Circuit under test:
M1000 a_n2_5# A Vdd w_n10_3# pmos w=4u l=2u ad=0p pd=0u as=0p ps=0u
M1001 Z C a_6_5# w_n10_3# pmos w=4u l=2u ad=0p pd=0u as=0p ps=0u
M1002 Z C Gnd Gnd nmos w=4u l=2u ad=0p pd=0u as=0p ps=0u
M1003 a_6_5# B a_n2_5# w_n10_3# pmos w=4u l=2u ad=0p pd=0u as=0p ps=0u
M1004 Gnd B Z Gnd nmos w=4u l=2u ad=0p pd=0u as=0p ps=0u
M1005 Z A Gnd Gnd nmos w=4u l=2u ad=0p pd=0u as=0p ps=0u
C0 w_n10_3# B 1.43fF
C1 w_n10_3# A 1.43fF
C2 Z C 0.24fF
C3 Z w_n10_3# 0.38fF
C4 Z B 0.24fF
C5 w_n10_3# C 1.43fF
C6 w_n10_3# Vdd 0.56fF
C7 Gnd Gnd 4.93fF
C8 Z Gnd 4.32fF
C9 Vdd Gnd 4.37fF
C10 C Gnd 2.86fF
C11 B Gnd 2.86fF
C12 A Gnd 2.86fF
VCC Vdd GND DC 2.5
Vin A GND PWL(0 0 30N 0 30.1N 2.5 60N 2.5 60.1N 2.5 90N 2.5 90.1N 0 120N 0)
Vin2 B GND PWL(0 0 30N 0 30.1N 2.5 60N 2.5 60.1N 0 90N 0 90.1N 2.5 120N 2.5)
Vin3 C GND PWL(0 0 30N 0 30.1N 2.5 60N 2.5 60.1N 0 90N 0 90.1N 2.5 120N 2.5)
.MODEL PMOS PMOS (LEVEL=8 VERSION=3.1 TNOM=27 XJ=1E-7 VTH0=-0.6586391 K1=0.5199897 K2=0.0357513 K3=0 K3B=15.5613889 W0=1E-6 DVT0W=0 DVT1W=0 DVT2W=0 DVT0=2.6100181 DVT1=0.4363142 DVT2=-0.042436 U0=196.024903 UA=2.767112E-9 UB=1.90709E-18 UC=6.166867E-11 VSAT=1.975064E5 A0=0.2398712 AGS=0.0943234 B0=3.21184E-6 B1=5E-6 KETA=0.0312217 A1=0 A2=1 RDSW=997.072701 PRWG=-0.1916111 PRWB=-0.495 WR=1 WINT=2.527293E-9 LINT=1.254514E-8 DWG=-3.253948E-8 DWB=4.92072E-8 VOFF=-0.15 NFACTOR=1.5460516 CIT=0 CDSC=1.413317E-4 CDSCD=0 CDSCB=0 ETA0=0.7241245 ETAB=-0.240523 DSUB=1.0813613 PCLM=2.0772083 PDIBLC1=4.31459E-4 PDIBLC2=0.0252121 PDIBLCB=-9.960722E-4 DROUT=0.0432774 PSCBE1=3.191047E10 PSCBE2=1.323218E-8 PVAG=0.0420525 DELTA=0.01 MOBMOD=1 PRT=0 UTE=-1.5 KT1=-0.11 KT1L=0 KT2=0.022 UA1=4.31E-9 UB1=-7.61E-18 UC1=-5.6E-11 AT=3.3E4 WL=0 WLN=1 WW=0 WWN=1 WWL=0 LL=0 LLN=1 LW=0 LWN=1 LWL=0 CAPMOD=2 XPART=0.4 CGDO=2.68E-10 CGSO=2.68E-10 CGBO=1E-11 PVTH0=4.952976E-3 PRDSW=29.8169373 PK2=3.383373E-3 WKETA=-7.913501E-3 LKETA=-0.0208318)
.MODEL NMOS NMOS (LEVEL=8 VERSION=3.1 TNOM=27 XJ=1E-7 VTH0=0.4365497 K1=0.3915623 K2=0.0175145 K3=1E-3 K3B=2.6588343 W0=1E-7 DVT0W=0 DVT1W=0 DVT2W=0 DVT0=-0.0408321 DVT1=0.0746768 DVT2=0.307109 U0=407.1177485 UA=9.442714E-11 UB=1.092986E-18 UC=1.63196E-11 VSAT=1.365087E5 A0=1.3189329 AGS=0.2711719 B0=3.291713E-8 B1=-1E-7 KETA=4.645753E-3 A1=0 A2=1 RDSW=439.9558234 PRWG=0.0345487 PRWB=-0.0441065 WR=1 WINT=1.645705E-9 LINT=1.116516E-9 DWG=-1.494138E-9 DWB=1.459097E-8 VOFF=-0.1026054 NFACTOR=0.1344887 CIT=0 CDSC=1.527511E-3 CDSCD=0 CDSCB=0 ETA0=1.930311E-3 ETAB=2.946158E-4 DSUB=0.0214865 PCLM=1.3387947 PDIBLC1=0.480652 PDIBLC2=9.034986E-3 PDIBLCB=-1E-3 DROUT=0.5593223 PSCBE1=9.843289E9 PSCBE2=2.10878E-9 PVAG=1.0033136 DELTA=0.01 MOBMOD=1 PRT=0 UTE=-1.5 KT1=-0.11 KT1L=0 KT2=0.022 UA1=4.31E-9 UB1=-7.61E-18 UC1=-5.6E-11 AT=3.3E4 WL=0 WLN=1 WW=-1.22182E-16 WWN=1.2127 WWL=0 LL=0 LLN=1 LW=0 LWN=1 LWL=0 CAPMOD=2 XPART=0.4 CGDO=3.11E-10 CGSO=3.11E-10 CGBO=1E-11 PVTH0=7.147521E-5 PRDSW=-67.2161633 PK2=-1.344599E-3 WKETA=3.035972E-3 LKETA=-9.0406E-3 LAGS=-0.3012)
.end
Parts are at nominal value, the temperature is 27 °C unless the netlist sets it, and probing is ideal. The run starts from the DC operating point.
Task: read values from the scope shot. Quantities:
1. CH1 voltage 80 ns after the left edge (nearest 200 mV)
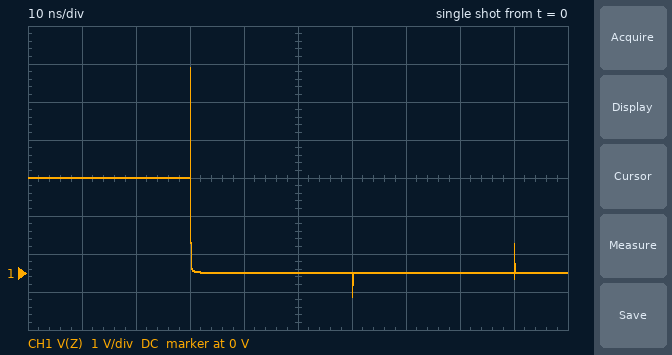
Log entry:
0 V
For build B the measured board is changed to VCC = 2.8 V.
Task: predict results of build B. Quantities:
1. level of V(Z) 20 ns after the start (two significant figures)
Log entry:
2.8 V
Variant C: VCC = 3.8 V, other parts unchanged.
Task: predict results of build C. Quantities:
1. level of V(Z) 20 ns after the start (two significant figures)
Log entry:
3.8 V
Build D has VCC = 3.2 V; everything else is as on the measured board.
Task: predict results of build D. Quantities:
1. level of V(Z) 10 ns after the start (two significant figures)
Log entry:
3.2 V
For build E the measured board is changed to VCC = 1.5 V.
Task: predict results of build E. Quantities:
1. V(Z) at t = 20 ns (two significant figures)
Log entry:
1.5 V
